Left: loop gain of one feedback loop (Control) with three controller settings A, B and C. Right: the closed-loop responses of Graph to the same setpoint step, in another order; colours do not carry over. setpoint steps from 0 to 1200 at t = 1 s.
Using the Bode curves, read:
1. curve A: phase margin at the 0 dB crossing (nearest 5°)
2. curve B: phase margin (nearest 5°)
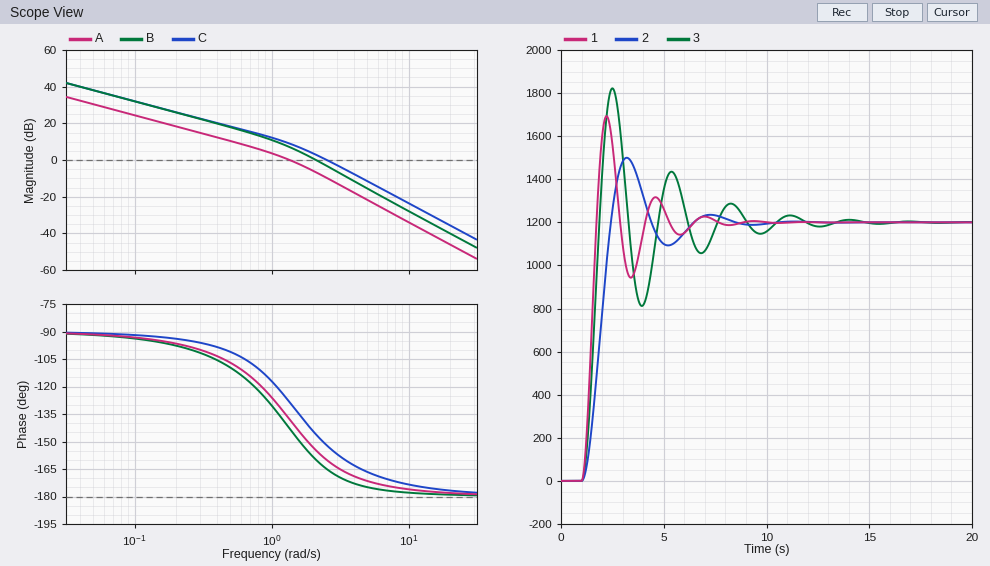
40°
20°
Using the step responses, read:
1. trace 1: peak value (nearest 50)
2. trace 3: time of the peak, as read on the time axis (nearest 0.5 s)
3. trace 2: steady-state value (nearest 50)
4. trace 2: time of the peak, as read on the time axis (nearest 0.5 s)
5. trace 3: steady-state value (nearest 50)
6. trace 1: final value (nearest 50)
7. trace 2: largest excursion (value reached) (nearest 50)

1700
2.5 s
1200
3.0 s
1200
1200
1500
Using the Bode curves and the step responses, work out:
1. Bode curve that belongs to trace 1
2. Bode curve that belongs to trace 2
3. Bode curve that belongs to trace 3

C
A
B
